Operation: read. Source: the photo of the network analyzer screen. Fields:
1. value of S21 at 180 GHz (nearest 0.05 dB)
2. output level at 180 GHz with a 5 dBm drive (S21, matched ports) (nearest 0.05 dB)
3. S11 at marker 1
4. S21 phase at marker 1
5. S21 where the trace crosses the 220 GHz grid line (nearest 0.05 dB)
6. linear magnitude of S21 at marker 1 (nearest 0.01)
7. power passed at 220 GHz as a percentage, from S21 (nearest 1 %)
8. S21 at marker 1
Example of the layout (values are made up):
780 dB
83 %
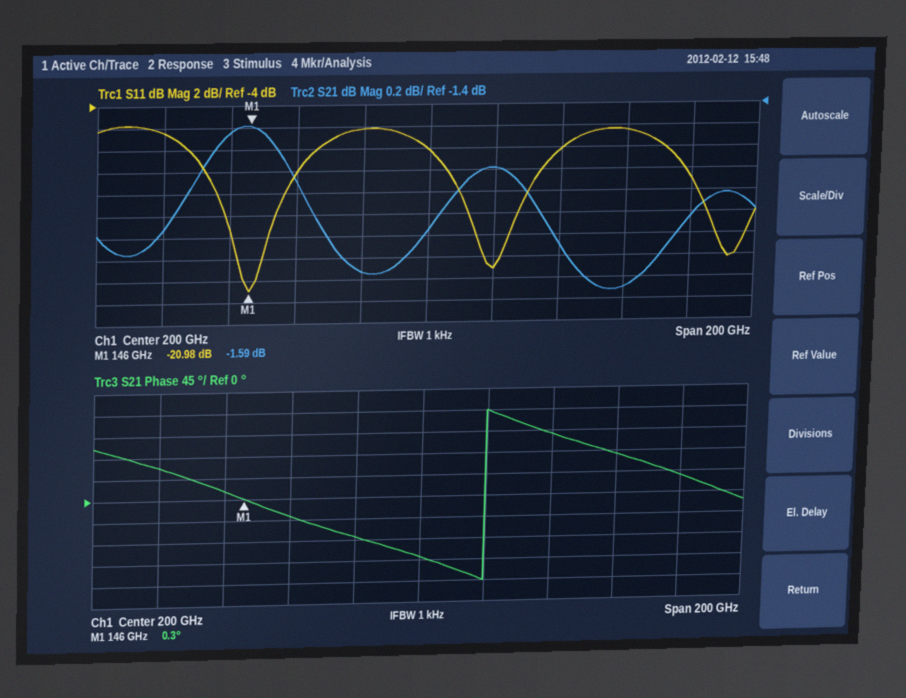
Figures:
-2.95 dB
2.05 dBm
-20.98 dB
0.3°
-2.00 dB
0.83
63 %
-1.59 dB
